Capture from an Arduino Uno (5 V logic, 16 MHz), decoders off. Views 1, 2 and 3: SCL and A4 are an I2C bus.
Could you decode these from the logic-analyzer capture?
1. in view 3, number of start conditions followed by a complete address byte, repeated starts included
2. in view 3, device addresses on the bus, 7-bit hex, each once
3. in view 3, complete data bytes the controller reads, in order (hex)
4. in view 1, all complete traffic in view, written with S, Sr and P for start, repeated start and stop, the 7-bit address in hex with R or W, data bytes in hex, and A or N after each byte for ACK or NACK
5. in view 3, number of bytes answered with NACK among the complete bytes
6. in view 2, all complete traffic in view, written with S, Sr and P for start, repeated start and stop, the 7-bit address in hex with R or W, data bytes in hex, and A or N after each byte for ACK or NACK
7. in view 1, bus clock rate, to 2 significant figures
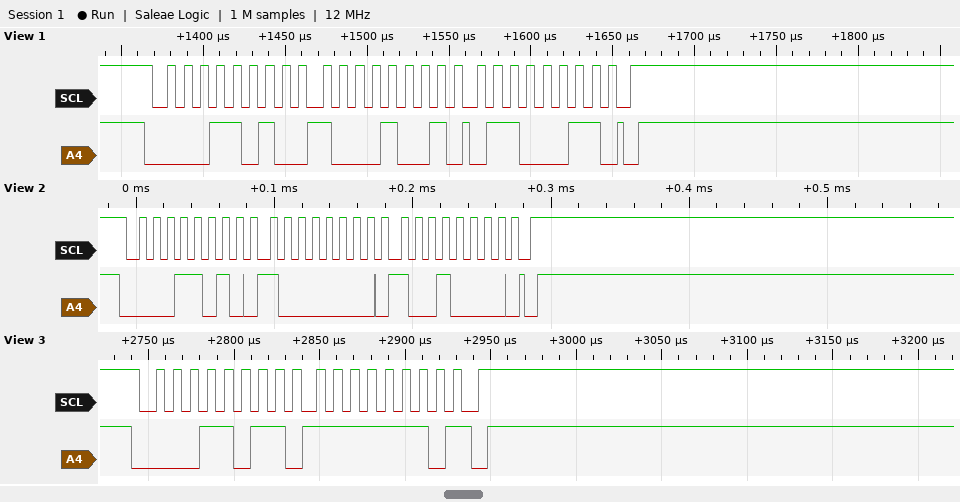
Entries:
1
0x0D
FE
S 0DW A 89 A 63 A P
1
S 0DW A 80 A 90 A P
100 kHz
